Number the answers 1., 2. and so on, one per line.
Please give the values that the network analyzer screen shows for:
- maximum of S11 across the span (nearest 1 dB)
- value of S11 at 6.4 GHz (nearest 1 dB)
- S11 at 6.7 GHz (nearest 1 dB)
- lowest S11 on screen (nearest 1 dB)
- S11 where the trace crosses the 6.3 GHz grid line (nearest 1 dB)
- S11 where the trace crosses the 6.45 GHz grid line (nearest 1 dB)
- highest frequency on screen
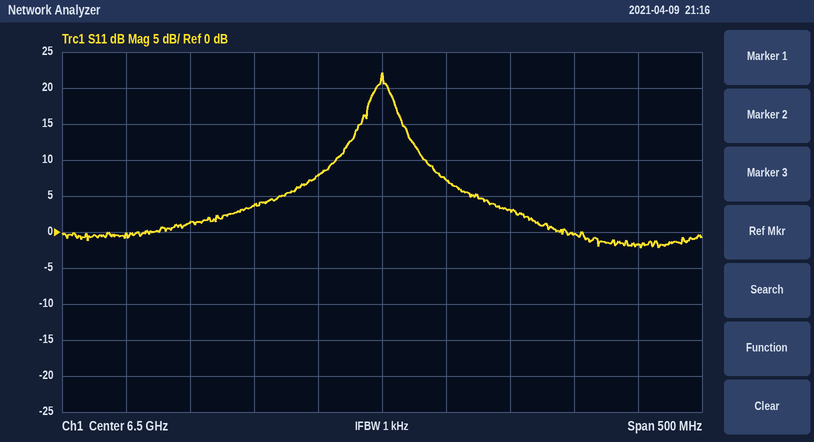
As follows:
1. 22 dB
2. 4 dB
3. -2 dB
4. -2 dB
5. 0 dB
6. 8 dB
7. 6.75 GHz
